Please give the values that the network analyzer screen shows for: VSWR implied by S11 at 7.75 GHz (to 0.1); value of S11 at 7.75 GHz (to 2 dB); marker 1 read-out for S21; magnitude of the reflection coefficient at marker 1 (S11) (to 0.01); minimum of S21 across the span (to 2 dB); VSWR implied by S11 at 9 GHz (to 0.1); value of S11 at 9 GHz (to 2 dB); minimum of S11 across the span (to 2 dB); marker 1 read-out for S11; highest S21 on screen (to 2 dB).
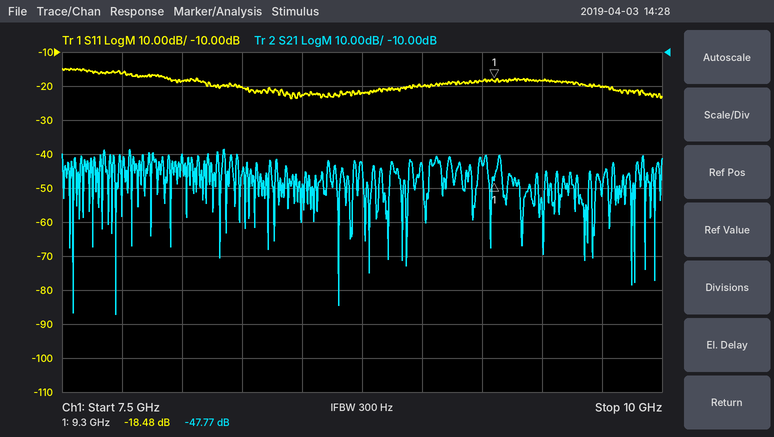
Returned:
1.4
-16 dB
-47.77 dB
0.12
-88 dB
1.2
-20 dB
-24 dB
-18.48 dB
-38 dB
